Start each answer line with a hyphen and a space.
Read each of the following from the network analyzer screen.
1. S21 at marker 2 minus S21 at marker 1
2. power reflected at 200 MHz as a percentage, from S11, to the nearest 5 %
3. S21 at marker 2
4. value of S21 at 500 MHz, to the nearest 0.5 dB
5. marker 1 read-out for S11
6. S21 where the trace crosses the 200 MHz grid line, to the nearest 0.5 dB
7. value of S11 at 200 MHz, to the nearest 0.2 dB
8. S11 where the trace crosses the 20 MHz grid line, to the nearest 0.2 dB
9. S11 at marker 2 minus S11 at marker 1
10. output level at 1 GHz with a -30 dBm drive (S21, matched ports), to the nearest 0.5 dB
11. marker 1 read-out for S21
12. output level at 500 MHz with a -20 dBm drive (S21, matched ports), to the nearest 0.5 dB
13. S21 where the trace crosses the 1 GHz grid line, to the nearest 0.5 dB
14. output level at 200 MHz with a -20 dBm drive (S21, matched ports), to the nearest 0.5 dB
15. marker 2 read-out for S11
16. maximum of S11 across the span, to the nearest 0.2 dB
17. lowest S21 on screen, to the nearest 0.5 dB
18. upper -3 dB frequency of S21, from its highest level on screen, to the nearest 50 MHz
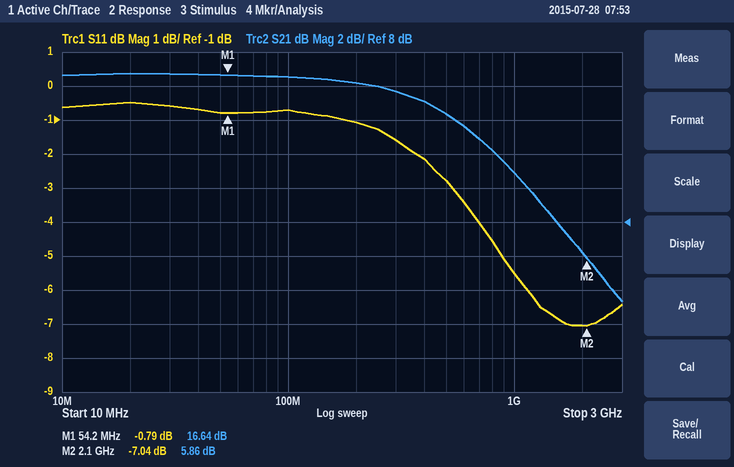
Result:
- -10.78 dB
- 80 %
- 5.86 dB
- 14.5 dB
- -0.79 dB
- 16.0 dB
- -1.0 dB
- -0.4 dB
- -6.25 dB
- -19.0 dBm
- 16.64 dB
- -5.5 dBm
- 11.0 dB
- -4.0 dBm
- -7.04 dB
- -0.4 dB
- 3.5 dB
- 600 MHz
